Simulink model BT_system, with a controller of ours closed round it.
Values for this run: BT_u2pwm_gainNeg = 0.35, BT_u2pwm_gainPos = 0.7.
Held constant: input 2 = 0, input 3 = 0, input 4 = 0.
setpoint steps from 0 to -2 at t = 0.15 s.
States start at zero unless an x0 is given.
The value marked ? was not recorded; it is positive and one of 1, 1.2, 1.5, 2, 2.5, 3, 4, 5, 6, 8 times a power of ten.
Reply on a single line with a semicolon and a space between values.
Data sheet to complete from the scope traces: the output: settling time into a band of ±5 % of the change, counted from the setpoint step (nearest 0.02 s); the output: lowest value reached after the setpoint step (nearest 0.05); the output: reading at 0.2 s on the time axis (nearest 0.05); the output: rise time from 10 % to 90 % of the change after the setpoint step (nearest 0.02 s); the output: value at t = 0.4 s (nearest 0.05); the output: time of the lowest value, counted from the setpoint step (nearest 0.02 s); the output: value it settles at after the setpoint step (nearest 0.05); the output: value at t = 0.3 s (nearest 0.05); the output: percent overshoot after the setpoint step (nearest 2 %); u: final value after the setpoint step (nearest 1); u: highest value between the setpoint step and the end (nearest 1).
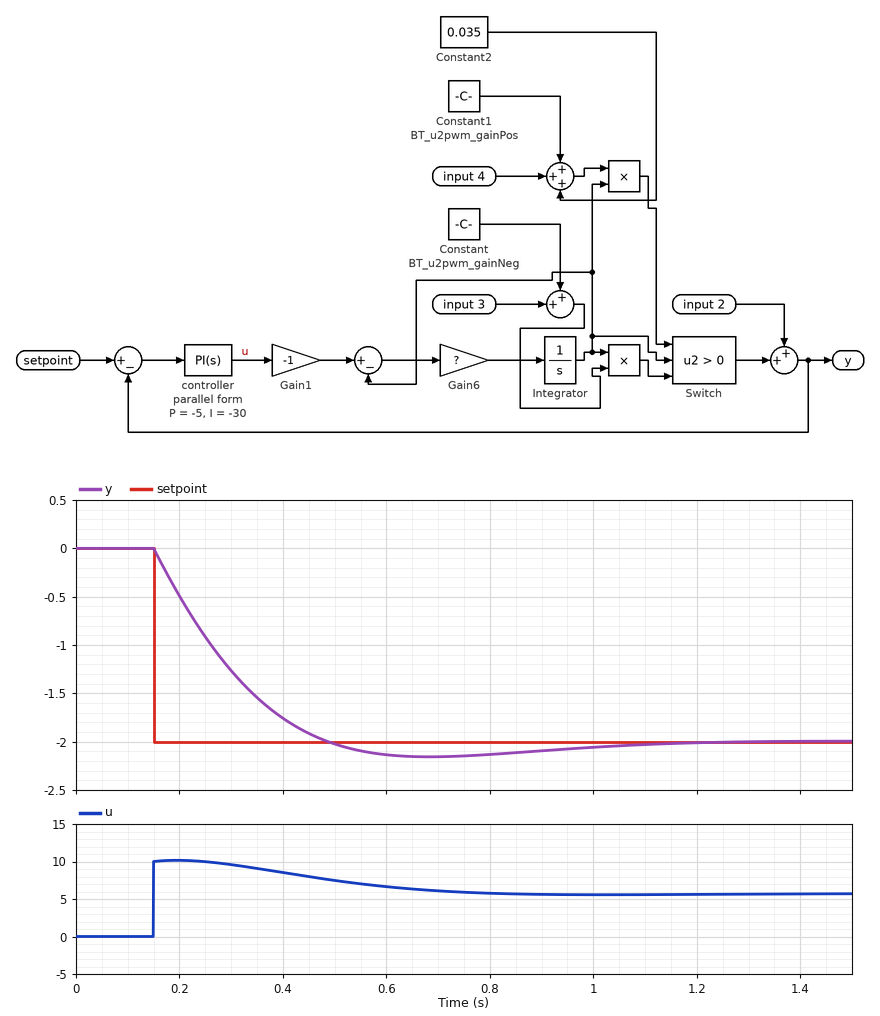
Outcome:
0.74 s; -2.15; -0.50; 0.24 s; -1.75; 0.54 s; -2.00; -1.25; 8 %; 6; 10
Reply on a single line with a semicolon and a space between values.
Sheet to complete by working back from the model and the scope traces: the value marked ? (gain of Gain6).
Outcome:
3
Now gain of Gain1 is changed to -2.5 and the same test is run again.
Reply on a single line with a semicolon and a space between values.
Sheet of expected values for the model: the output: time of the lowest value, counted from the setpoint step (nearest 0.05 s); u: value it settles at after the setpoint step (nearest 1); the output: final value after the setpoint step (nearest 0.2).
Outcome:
0.30 s; 2; -2.0
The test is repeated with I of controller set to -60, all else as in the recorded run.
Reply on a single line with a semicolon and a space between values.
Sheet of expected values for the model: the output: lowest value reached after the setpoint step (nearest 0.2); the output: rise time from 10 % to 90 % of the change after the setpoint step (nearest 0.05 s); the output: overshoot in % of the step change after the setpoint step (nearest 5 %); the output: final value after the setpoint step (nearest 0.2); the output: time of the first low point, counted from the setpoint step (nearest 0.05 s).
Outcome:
-2.4; 0.15 s; 20 %; -2.0; 0.35 s
